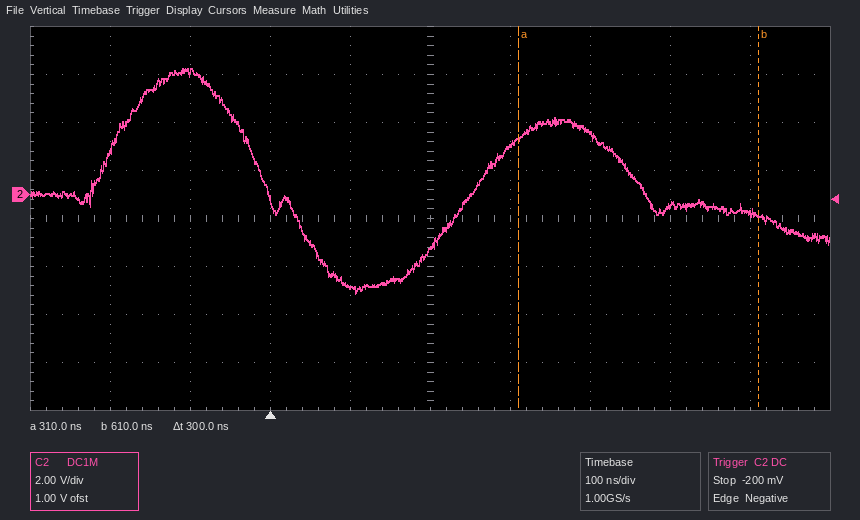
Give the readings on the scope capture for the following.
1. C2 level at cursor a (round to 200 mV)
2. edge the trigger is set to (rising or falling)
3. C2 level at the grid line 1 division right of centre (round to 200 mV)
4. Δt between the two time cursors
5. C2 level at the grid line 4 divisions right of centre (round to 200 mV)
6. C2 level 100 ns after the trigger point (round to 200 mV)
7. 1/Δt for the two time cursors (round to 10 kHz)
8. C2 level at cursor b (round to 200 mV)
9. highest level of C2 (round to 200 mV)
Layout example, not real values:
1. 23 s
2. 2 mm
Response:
1. 2.4 V
2. falling
3. 2.0 V
4. 300 ns
5. -800 mV
6. -3.8 V
7. 3.33 MHz
8. -800 mV
9. 5.2 V
